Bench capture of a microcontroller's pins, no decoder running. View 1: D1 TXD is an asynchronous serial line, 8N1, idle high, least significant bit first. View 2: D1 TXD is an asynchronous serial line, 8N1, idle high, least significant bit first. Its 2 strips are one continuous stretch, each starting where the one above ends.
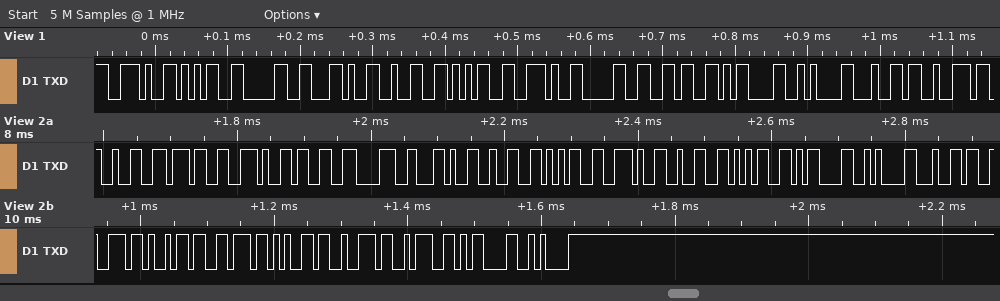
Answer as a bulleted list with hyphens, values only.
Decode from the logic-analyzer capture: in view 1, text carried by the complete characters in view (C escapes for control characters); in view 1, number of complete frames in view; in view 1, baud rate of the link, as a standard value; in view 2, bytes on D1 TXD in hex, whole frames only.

- ".50,25.06\r\ndr"
- 13
- 115200 baud
- 32 37 2E 33 38 2C 32 35 2E 32 35 0D 0A 64 72 69 76 65 72 3A 0D 0A
